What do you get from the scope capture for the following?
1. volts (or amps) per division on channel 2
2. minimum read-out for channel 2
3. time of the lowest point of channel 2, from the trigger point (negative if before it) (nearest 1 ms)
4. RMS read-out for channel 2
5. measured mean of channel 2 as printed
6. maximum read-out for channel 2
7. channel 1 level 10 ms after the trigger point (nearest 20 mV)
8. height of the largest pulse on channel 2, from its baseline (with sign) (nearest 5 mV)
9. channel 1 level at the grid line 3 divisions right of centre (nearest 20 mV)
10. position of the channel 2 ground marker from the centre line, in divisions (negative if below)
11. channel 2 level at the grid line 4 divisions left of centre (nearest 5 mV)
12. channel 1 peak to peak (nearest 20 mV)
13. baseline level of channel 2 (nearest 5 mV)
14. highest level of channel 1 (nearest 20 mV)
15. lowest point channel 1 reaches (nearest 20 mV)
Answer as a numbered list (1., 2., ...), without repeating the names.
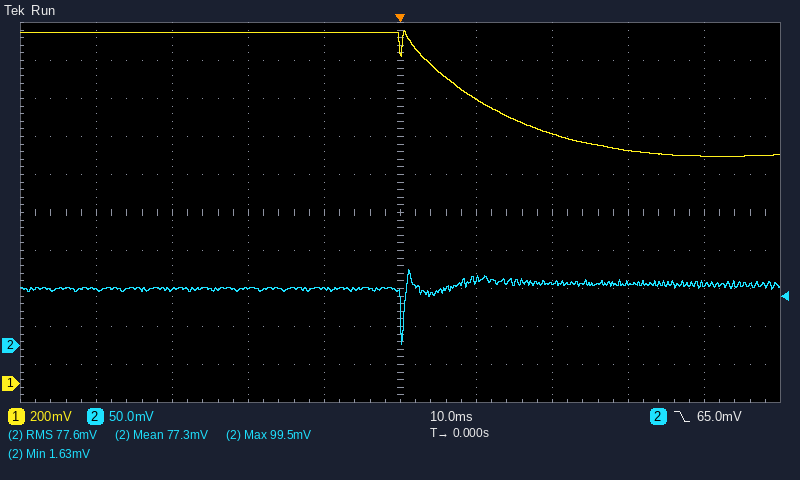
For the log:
1. 50 mV
2. 1.63 mV
3. 0 ms
4. 77.6 mV
5. 77.3 mV
6. 99.5 mV
7. 1.50 V
8. -75 mV
9. 1.22 V
10. -3.5 div
11. 75 mV
12. 660 mV
13. 75 mV
14. 1.86 V
15. 1.20 V
